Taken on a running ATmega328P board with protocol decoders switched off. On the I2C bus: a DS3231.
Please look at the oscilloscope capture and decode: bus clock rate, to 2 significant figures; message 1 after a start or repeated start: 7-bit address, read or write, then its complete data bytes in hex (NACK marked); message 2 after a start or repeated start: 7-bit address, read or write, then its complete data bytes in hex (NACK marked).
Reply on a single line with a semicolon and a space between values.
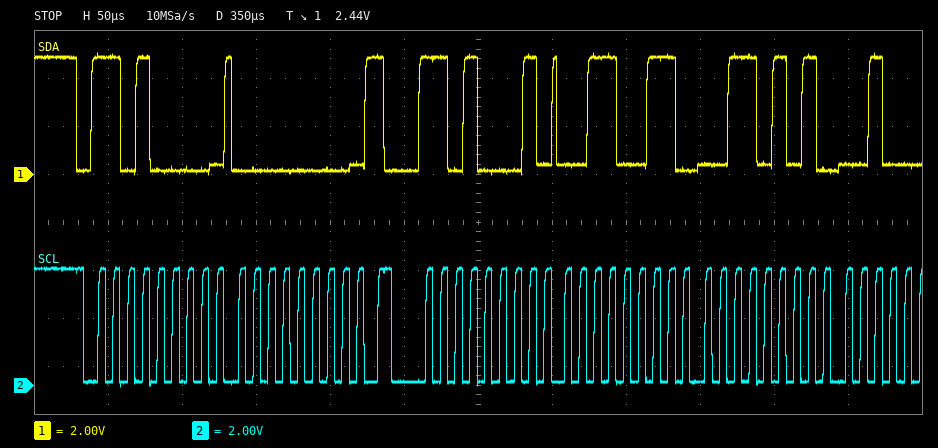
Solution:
100 kHz; 0x68 write: 00; 0x68 read: 33 35
